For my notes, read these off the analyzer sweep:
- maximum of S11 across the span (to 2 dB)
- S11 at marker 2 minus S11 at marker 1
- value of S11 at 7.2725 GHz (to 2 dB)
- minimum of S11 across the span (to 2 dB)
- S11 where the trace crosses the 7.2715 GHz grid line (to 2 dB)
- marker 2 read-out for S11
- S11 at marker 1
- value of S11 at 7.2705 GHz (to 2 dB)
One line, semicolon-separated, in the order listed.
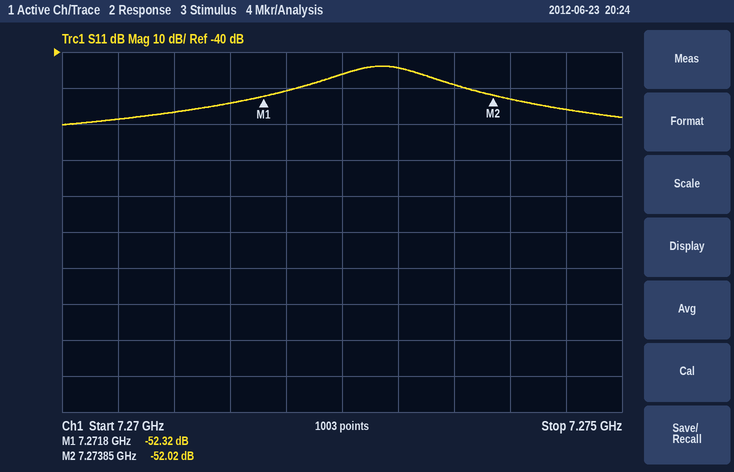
-44 dB; 0.30 dB; -46 dB; -60 dB; -54 dB; -52.02 dB; -52.32 dB; -58 dB
